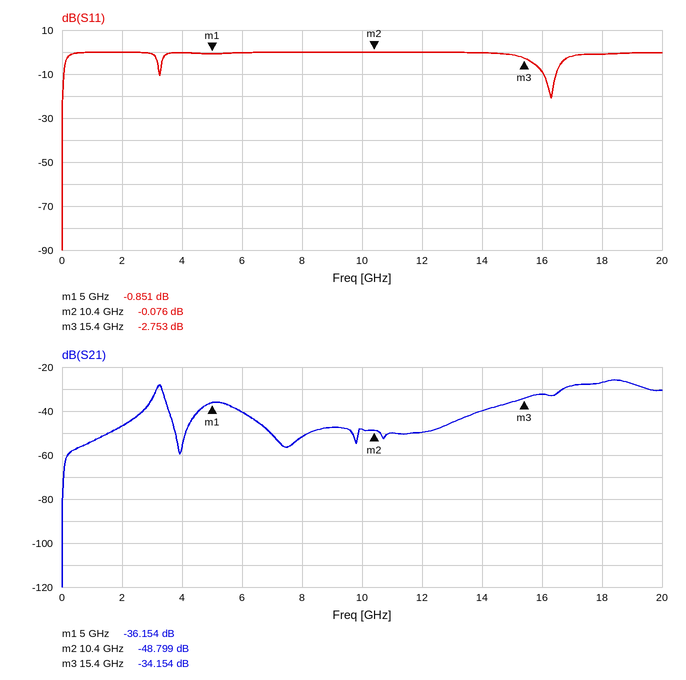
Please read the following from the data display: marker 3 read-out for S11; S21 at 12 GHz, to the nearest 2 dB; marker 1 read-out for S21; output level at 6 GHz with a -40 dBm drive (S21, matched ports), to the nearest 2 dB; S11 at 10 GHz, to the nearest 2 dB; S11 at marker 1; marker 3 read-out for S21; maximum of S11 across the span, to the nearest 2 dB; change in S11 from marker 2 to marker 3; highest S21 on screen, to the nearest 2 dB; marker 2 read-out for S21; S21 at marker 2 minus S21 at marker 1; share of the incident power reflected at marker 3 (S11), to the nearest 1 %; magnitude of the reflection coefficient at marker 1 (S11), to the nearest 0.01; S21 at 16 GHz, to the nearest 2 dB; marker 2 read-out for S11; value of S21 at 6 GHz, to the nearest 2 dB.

-2.753 dB
-50 dB
-36.154 dB
-80 dBm
0 dB
-0.851 dB
-34.154 dB
0 dB
-2.677 dB
-26 dB
-48.799 dB
-12.645 dB
53 %
0.91
-32 dB
-0.076 dB
-40 dB
